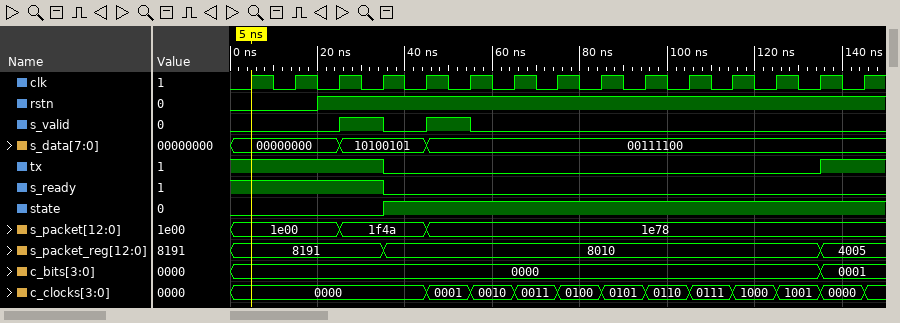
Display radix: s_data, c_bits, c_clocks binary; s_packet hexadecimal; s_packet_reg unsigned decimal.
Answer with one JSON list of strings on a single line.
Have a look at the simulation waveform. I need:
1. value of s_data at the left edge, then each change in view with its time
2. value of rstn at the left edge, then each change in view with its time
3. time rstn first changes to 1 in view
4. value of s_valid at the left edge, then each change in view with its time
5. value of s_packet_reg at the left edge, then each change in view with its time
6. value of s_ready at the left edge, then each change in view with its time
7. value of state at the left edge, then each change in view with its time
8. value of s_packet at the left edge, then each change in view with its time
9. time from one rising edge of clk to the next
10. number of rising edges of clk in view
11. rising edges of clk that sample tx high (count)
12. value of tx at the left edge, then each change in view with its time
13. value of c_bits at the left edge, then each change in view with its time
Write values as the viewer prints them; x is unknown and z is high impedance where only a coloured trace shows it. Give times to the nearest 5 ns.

["00000000, 10100101 at 25 ns, 00111100 at 45 ns", "0, 1 at 20 ns", "20 ns", "0, 1 at 25 ns, 0 at 35 ns, 1 at 45 ns, 0 at 55 ns", "8191, 8010 at 35 ns, 4005 at 135 ns", "1, 0 at 35 ns", "0, 1 at 35 ns", "1e00, 1f4a at 25 ns, 1e78 at 45 ns", "10 ns", "15", "5", "1, 0 at 35 ns, 1 at 135 ns", "0000, 0001 at 135 ns"]
